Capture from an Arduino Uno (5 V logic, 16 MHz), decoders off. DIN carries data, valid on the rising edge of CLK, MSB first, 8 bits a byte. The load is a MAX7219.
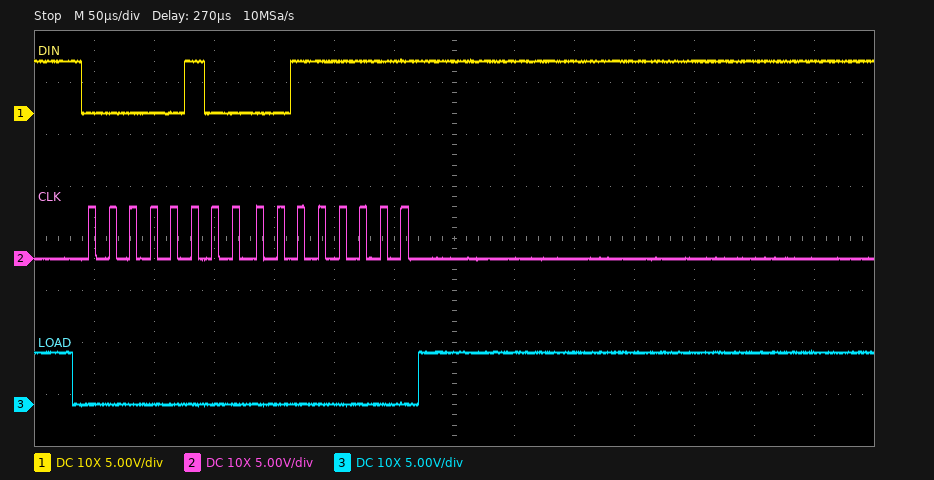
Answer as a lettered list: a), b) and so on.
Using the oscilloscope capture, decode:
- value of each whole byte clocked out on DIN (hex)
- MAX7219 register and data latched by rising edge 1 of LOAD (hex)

a) 04 3F
b) register 0x4, data 0x3F
